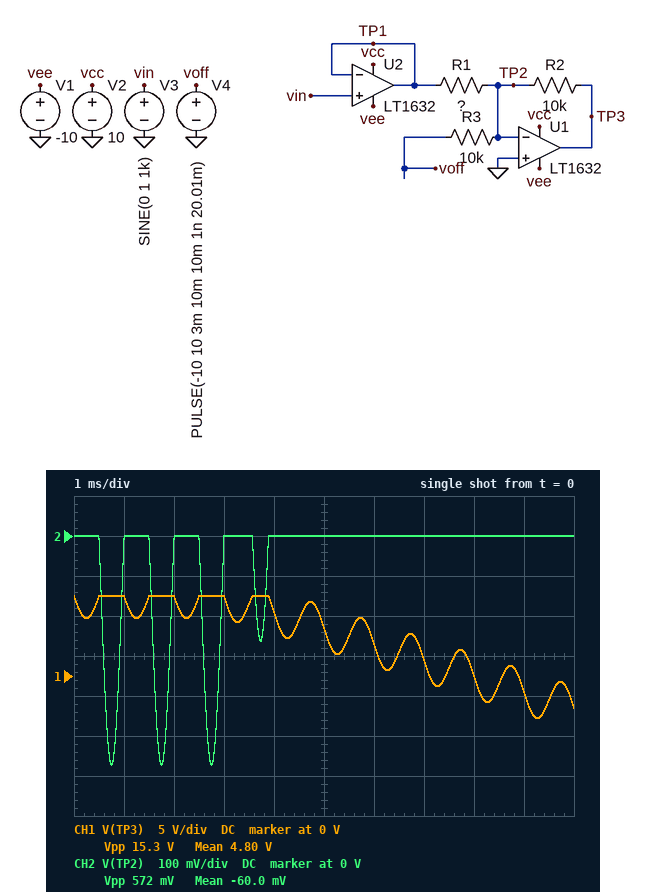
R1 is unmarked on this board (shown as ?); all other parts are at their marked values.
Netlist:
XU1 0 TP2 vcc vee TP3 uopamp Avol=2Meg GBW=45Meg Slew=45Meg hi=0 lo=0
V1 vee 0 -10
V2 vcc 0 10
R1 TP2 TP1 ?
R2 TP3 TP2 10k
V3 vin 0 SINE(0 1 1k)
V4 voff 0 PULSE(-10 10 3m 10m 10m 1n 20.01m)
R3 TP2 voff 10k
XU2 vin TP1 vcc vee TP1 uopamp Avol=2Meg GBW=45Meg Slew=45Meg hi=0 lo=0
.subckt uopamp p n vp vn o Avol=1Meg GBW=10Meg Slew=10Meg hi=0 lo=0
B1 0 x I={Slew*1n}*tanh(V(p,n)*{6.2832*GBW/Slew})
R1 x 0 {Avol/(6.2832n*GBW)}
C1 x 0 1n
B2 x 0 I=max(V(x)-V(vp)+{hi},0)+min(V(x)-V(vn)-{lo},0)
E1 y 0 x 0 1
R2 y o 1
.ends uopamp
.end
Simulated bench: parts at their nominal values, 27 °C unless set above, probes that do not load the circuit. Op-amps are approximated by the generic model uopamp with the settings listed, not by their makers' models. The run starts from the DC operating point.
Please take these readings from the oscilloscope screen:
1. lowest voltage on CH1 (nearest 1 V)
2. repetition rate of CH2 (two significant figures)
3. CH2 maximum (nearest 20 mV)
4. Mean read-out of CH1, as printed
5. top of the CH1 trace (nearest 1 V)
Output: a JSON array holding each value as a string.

["-5 V", "1.0 kHz", "0 V", "4.80 V", "10 V"]
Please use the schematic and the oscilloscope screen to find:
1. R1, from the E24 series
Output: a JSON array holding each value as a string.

["3.6 kΩ"]
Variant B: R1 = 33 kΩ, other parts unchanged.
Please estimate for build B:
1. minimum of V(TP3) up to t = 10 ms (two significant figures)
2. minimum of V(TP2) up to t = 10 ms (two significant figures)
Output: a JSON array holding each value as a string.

["-4.0 V", "-120 mV"]
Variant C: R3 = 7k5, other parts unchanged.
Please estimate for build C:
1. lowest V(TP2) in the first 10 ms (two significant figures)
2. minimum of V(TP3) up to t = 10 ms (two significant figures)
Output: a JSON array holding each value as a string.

["-1.2 V", "-6.1 V"]
